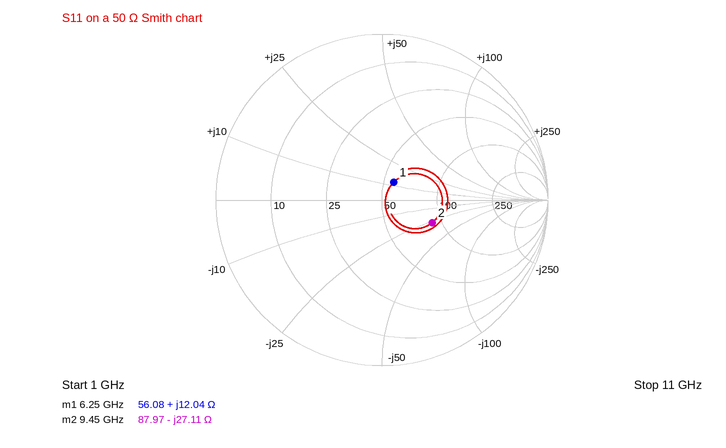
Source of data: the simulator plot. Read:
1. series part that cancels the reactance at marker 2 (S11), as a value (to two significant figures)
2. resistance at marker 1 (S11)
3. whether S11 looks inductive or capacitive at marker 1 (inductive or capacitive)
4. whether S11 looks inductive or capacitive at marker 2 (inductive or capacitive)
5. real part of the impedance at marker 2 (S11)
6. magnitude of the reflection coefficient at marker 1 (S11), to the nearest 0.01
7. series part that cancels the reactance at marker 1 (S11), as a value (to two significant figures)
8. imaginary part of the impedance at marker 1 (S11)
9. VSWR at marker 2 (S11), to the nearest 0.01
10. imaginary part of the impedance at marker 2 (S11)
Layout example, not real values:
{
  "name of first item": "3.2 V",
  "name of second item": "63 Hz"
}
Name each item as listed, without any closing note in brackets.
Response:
{
  "series part that cancels the reactance at marker 2 (S11), as a value": "460 pH",
  "resistance at marker 1": "56.08 Ω",
  "whether S11 looks inductive or capacitive at marker 1": "inductive",
  "whether S11 looks inductive or capacitive at marker 2": "capacitive",
  "real part of the impedance at marker 2": "87.97 Ω",
  "magnitude of the reflection coefficient at marker 1 (S11), to the nearest 0.01": "0.13",
  "series part that cancels the reactance at marker 1 (S11), as a value": "2.1 pF",
  "imaginary part of the impedance at marker 1": "+12.04 Ω",
  "VSWR at marker 2 (S11), to the nearest 0.01": "1.99",
  "imaginary part of the impedance at marker 2": "-27.11 Ω"
}
